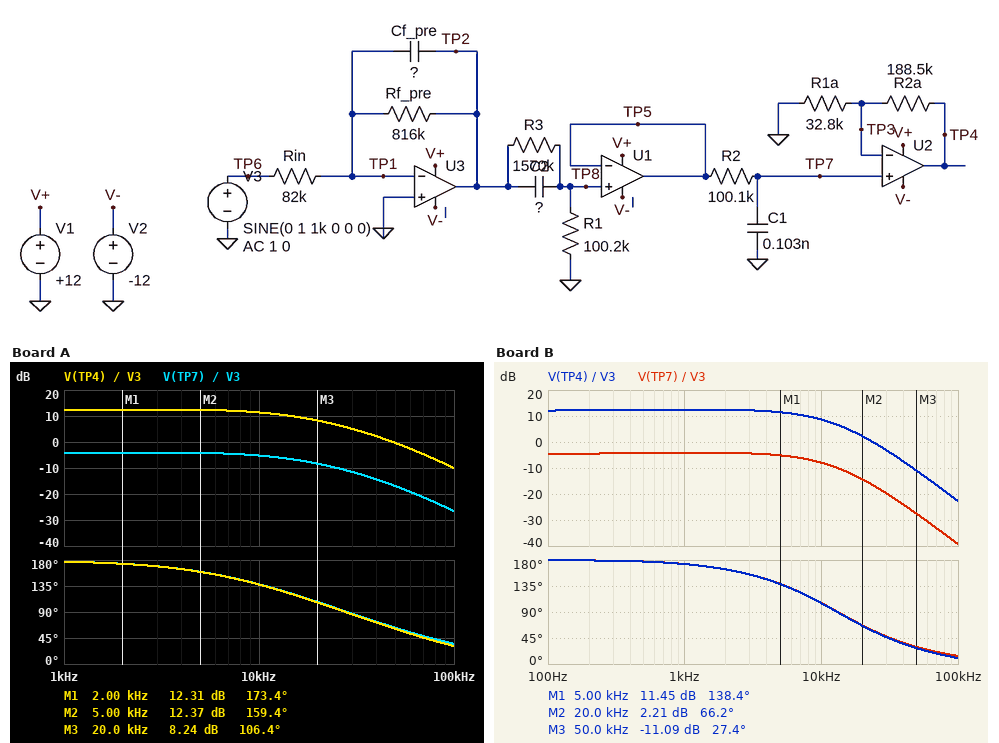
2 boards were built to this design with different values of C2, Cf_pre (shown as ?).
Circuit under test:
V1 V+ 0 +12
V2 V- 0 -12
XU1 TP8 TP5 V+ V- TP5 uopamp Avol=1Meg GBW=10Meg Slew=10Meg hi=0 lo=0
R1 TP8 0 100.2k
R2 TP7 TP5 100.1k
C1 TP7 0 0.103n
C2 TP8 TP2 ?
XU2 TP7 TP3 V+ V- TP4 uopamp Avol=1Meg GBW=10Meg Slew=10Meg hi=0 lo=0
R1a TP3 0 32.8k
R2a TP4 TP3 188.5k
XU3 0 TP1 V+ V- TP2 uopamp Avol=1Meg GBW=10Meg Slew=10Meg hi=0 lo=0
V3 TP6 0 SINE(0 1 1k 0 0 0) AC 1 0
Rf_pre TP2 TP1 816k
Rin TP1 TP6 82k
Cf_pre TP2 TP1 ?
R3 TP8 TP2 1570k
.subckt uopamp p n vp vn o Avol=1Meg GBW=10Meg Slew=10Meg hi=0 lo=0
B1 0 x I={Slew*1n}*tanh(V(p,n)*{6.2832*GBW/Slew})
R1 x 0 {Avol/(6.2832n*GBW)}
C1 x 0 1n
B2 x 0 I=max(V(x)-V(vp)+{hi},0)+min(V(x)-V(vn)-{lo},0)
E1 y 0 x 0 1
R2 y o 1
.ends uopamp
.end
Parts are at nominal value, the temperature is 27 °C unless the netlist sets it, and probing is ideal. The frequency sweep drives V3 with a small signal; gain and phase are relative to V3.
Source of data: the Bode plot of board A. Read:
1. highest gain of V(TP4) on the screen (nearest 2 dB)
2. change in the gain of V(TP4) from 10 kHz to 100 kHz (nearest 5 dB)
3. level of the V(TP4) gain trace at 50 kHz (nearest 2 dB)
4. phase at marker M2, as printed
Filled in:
12 dB
-20 dB
0 dB
159.4 deg
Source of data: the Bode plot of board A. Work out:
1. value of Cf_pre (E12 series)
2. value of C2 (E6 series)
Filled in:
56 pF
33 pF
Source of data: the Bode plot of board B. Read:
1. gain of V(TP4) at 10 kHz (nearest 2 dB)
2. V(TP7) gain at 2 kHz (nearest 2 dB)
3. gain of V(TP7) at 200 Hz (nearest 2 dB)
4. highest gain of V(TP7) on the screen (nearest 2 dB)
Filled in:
8 dB
-4 dB
-4 dB
-4 dB
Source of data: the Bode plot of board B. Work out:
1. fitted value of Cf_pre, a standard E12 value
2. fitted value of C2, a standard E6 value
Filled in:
270 pF
150 pF
